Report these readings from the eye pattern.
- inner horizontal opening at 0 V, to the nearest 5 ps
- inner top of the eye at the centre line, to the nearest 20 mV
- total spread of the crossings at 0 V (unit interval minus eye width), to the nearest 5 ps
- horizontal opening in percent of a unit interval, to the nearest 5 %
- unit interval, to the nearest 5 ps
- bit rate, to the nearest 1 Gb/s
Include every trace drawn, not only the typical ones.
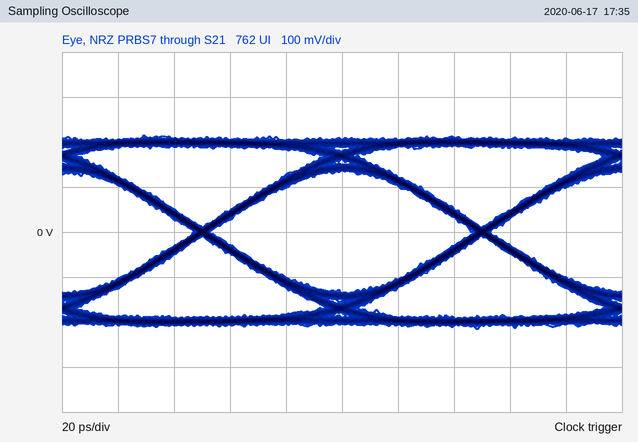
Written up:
95 ps
140 mV
5 ps
95 %
100 ps
10 Gb/s
